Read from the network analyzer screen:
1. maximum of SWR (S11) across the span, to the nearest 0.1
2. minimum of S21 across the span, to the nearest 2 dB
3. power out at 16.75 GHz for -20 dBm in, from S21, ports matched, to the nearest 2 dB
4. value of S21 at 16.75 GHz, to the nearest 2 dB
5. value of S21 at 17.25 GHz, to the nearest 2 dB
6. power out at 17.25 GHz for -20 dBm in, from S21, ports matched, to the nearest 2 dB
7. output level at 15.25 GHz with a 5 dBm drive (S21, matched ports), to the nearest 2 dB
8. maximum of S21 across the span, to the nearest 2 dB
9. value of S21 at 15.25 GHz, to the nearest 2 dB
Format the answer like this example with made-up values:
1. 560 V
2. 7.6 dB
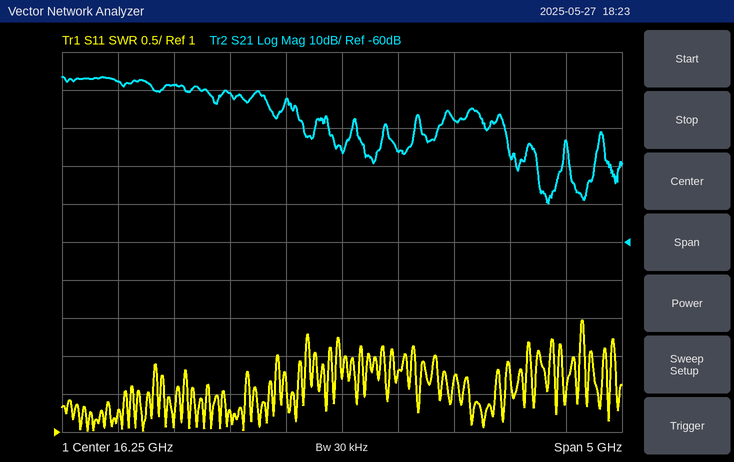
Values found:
1. 2.5
2. -50 dB
3. -56 dBm
4. -36 dB
5. -28 dB
6. -48 dBm
7. -16 dBm
8. -16 dB
9. -20 dB
